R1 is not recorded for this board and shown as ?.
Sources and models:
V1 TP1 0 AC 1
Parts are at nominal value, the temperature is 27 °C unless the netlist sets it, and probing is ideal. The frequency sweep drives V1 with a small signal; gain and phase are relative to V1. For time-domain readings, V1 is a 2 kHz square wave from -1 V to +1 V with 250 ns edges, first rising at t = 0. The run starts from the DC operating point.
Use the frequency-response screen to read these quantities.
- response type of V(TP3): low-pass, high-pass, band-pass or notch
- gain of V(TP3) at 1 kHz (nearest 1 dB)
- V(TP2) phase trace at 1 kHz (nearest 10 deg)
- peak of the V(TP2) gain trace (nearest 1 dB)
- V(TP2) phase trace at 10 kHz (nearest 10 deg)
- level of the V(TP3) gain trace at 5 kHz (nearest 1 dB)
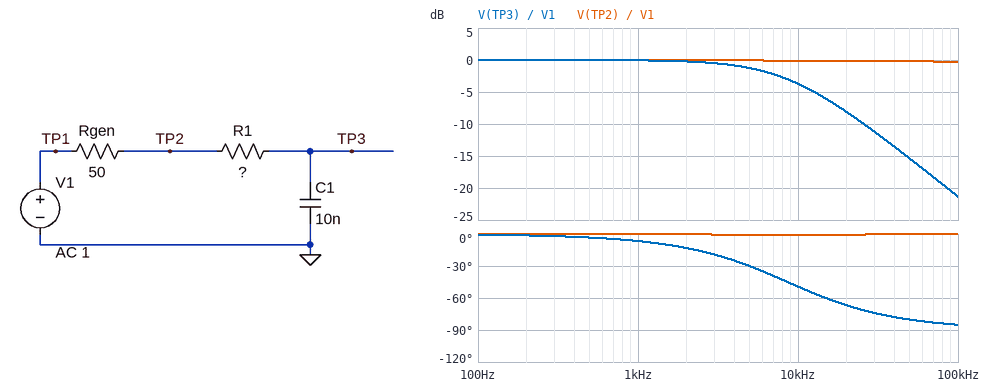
low-pass
0 dB
0 deg
0 dB
0 deg
-1 dB
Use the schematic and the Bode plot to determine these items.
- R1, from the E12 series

1.8 kΩ
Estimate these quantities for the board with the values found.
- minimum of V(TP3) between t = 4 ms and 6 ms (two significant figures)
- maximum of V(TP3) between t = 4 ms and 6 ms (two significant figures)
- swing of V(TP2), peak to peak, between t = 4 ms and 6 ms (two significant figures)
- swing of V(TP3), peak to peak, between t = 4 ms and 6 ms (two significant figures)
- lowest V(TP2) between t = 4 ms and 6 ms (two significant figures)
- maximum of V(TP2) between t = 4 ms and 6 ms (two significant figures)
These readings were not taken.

-1.0 V
1.0 V
2.0 V
2.0 V
-1.0 V
1.0 V
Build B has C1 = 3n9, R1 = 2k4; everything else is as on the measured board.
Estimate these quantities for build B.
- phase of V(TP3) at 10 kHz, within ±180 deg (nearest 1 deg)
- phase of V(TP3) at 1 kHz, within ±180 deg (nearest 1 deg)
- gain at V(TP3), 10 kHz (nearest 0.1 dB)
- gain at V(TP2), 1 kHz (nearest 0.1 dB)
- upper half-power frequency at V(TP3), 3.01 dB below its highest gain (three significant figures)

-31 deg
-3 deg
-1.3 dB
0 dB
16.7 kHz
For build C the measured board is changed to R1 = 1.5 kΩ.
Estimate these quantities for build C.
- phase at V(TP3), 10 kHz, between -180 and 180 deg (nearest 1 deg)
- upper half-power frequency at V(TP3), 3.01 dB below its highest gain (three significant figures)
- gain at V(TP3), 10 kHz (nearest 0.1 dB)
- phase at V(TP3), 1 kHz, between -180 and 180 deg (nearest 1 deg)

-44 deg
10.3 kHz
-2.9 dB
-6 deg
